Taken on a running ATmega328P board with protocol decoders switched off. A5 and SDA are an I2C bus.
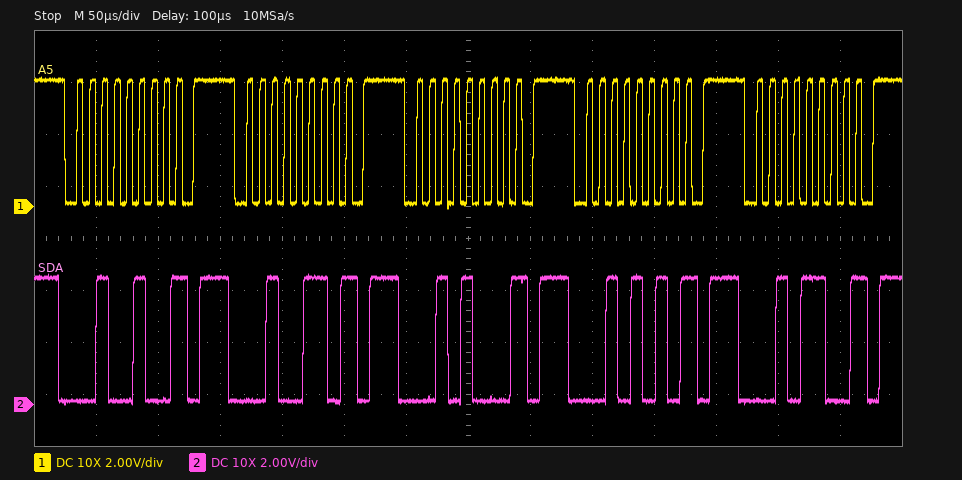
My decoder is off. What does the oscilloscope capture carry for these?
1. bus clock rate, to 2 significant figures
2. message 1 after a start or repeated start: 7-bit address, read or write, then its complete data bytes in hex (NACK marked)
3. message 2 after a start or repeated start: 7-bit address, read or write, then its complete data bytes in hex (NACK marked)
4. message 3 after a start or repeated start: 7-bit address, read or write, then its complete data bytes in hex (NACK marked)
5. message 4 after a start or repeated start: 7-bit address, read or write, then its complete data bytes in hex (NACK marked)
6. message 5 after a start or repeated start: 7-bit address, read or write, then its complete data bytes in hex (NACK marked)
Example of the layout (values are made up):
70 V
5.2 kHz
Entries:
100 kHz
0x12 write NACK
0x13 write NACK
0x14 write NACK
0x15 write NACK
0x16 write NACK
